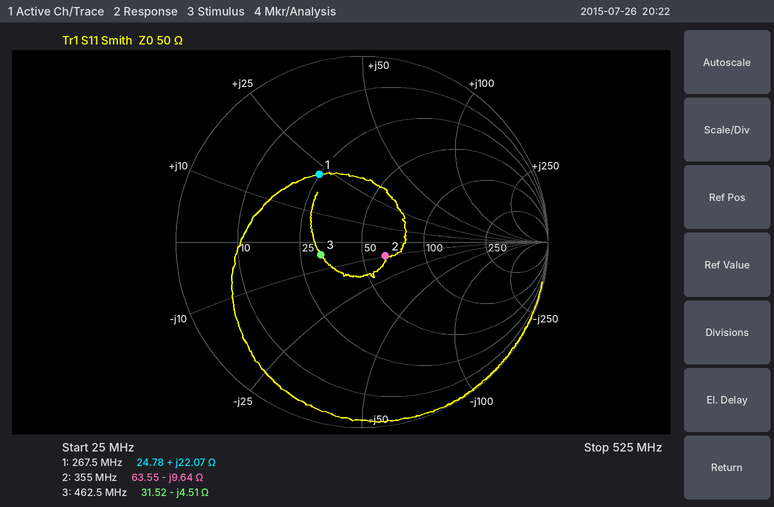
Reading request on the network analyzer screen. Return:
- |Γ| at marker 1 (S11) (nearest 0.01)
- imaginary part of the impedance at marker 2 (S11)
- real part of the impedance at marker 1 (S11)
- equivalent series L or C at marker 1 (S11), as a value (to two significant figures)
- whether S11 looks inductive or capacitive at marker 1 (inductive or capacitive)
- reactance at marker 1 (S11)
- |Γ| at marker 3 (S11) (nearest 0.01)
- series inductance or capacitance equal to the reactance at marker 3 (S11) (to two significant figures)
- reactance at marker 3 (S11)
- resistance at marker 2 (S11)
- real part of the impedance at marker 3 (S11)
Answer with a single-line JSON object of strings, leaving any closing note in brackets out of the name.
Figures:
{"|Γ| at marker 1 (S11)": "0.43", "imaginary part of the impedance at marker 2": "-9.64 Ω", "real part of the impedance at marker 1": "24.78 Ω", "equivalent series L or C at marker 1 (S11), as a value": "13 nH", "whether S11 looks inductive or capacitive at marker 1": "inductive", "reactance at marker 1": "+22.07 Ω", "|Γ| at marker 3 (S11)": "0.23", "series inductance or capacitance equal to the reactance at marker 3 (S11)": "76 pF", "reactance at marker 3": "-4.51 Ω", "resistance at marker 2": "63.55 Ω", "real part of the impedance at marker 3": "31.52 Ω"}
